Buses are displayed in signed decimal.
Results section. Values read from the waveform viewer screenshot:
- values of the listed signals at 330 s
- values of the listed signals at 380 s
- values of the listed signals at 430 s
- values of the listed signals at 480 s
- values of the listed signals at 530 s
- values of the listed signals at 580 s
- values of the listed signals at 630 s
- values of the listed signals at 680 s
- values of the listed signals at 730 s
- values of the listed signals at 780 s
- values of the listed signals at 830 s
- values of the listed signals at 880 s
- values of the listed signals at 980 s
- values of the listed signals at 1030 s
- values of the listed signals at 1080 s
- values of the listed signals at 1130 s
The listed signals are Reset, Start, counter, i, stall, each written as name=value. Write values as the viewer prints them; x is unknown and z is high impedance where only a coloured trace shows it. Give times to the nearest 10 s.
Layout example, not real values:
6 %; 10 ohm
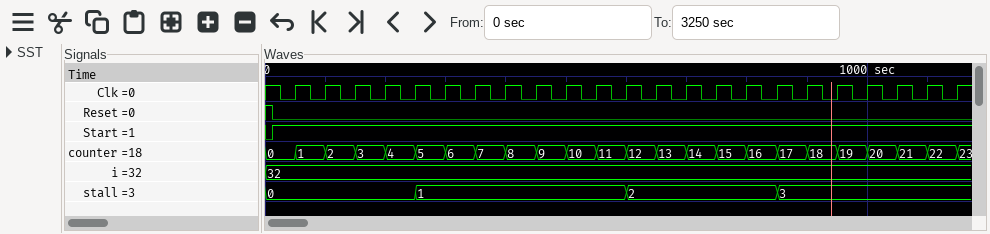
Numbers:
Reset=0, Start=1, counter=6, i=32, stall=1; Reset=0, Start=1, counter=7, i=32, stall=1; Reset=0, Start=1, counter=8, i=32, stall=1; Reset=0, Start=1, counter=9, i=32, stall=1; Reset=0, Start=1, counter=10, i=32, stall=1; Reset=0, Start=1, counter=11, i=32, stall=1; Reset=0, Start=1, counter=12, i=32, stall=2; Reset=0, Start=1, counter=13, i=32, stall=2; Reset=0, Start=1, counter=14, i=32, stall=2; Reset=0, Start=1, counter=15, i=32, stall=2; Reset=0, Start=1, counter=16, i=32, stall=2; Reset=0, Start=1, counter=17, i=32, stall=3; Reset=0, Start=1, counter=19, i=32, stall=3; Reset=0, Start=1, counter=20, i=32, stall=3; Reset=0, Start=1, counter=21, i=32, stall=3; Reset=0, Start=1, counter=22, i=32, stall=3
